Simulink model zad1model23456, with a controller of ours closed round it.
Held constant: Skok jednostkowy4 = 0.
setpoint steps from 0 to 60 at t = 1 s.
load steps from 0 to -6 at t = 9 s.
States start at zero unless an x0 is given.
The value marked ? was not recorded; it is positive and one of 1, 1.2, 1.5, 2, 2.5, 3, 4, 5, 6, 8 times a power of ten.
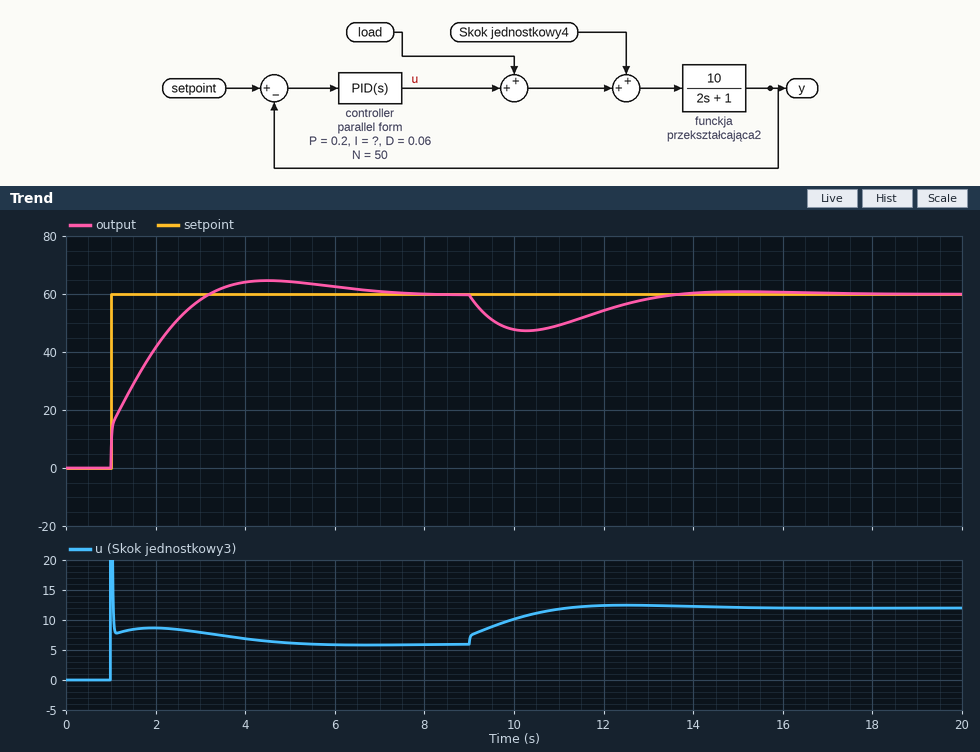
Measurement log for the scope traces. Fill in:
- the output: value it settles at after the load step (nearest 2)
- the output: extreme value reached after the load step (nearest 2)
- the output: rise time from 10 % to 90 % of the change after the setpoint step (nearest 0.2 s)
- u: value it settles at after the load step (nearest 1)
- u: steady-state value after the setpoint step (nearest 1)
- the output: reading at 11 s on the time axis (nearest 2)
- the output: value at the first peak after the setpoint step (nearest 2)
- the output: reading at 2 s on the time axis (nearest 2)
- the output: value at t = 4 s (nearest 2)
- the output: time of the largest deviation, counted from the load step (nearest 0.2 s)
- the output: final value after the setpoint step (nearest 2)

60
48
1.6 s
12
6
50
64
42
64
1.2 s
60
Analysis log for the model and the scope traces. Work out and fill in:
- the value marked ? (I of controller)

0.2
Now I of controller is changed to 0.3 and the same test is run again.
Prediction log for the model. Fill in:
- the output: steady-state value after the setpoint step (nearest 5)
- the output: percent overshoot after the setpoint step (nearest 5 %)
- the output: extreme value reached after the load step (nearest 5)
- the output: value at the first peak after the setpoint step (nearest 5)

60
15 %
50
70
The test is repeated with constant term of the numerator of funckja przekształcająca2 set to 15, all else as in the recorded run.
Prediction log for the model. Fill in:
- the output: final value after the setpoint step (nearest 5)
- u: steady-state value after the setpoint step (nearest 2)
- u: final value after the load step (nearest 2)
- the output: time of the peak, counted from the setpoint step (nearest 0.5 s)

60
4
10
3.0 s
